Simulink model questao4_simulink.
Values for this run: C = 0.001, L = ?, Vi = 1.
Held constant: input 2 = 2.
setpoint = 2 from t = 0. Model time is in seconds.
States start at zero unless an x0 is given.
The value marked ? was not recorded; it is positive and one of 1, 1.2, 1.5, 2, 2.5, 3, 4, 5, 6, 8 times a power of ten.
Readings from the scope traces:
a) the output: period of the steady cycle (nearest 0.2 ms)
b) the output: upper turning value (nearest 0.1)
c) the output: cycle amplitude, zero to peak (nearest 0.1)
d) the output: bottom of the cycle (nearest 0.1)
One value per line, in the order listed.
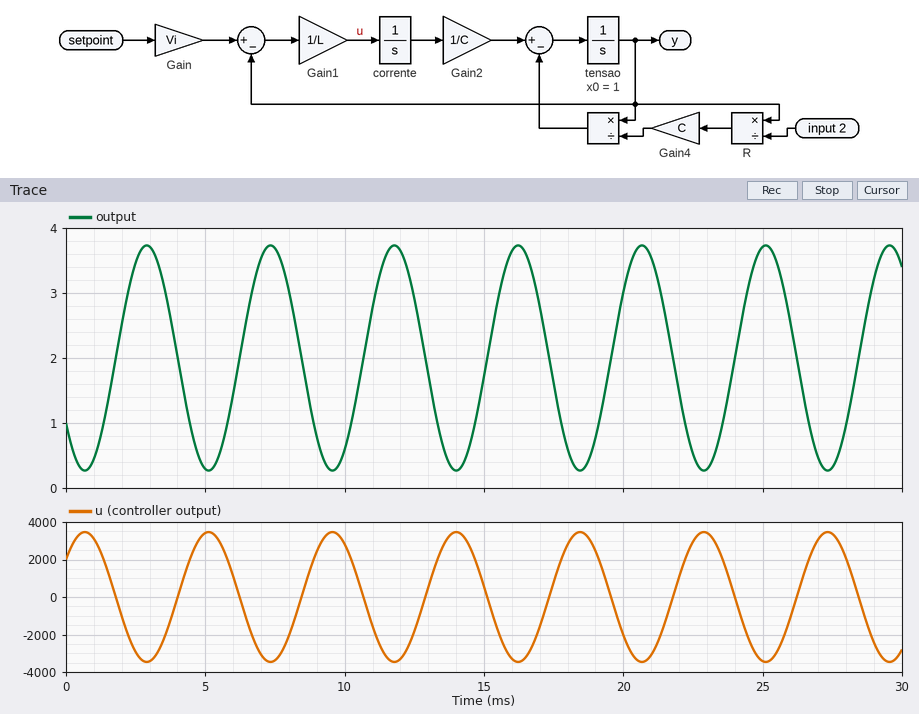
4.4 ms
3.7
1.7
0.3
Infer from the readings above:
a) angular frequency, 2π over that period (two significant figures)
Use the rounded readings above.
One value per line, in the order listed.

1.4 rad/ms
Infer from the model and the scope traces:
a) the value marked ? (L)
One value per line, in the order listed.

0.0005
